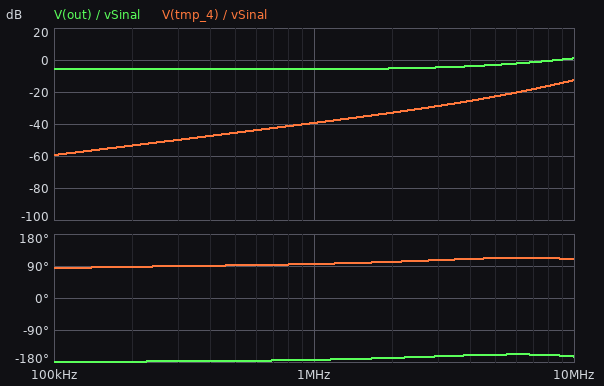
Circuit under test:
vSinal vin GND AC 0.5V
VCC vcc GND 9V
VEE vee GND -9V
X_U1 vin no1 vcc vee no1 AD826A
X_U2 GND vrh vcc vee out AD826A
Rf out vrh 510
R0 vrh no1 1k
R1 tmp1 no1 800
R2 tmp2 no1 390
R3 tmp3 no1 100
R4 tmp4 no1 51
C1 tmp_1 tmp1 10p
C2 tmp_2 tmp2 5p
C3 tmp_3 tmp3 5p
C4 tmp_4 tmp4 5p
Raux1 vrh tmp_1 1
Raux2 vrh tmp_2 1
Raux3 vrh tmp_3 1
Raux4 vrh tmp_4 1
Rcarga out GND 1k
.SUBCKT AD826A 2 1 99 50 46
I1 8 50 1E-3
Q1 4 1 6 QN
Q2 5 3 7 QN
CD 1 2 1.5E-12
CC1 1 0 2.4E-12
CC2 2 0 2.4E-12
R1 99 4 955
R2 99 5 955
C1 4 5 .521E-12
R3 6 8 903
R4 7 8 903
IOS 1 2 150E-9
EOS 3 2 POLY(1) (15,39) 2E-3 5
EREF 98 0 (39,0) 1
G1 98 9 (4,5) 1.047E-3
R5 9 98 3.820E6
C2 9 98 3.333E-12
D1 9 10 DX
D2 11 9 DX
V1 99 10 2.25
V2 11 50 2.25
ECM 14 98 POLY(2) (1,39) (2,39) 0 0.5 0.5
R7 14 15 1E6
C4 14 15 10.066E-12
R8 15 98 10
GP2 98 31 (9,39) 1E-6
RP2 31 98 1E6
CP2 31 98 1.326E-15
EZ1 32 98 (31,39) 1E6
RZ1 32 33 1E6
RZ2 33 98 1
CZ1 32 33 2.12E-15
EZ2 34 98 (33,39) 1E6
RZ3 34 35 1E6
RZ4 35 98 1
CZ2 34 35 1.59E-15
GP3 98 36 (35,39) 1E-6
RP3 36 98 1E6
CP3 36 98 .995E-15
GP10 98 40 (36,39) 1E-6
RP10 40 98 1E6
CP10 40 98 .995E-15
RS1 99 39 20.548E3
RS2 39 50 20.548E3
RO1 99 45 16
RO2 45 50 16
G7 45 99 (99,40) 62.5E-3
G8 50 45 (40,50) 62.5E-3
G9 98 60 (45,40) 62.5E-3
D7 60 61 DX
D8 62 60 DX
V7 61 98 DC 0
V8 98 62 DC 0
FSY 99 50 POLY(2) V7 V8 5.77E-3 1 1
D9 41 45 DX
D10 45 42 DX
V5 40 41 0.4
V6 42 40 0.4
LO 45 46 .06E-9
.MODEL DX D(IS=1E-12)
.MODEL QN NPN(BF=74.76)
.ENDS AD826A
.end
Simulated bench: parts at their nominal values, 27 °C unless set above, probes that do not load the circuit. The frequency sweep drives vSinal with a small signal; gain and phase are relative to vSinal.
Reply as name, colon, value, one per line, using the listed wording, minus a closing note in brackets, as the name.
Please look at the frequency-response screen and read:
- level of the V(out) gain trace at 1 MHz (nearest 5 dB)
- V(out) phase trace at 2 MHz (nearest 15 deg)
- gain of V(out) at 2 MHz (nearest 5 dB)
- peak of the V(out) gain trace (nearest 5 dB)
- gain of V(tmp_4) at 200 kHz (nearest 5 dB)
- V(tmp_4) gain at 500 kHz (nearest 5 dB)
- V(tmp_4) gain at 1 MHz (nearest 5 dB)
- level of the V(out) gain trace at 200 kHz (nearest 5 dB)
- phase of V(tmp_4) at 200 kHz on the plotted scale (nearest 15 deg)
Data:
level of the V(out) gain trace at 1 MHz: -5 dB
V(out) phase trace at 2 MHz: -165 deg
gain of V(out) at 2 MHz: -5 dB
peak of the V(out) gain trace: 0 dB
gain of V(tmp_4) at 200 kHz: -55 dB
V(tmp_4) gain at 500 kHz: -45 dB
V(tmp_4) gain at 1 MHz: -40 dB
level of the V(out) gain trace at 200 kHz: -5 dB
phase of V(tmp_4) at 200 kHz on the plotted scale: 90 deg
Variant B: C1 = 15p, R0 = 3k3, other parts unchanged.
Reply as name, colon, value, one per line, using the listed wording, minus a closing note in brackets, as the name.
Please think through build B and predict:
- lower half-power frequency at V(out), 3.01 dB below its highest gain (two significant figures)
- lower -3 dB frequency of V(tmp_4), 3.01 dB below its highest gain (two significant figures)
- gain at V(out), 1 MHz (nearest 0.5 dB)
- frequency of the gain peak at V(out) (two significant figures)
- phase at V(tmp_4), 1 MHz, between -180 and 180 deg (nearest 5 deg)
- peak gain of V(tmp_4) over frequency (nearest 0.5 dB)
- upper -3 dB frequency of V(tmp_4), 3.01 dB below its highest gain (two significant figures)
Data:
lower half-power frequency at V(out), 3.01 dB below its highest gain: 14 MHz
lower -3 dB frequency of V(tmp_4), 3.01 dB below its highest gain: 19 MHz
gain at V(out), 1 MHz: -14.5 dB
frequency of the gain peak at V(out): 23 MHz
phase at V(tmp_4), 1 MHz, between -180 and 180 deg: 120 deg
peak gain of V(tmp_4) over frequency: 0.5 dB
upper -3 dB frequency of V(tmp_4), 3.01 dB below its highest gain: 71 MHz
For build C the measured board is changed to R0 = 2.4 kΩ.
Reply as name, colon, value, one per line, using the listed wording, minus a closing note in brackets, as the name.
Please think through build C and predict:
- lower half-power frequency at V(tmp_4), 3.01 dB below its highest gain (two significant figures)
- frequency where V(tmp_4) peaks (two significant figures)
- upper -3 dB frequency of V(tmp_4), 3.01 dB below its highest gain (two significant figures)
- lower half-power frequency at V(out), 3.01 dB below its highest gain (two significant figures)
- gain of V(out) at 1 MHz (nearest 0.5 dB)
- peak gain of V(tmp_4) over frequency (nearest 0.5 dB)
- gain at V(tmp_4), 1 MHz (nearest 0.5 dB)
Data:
lower half-power frequency at V(tmp_4), 3.01 dB below its highest gain: 19 MHz
frequency where V(tmp_4) peaks: 28 MHz
upper -3 dB frequency of V(tmp_4), 3.01 dB below its highest gain: 65 MHz
lower half-power frequency at V(out), 3.01 dB below its highest gain: 15 MHz
gain of V(out) at 1 MHz: -13.0 dB
peak gain of V(tmp_4) over frequency: 1.0 dB
gain at V(tmp_4), 1 MHz: -46.5 dB
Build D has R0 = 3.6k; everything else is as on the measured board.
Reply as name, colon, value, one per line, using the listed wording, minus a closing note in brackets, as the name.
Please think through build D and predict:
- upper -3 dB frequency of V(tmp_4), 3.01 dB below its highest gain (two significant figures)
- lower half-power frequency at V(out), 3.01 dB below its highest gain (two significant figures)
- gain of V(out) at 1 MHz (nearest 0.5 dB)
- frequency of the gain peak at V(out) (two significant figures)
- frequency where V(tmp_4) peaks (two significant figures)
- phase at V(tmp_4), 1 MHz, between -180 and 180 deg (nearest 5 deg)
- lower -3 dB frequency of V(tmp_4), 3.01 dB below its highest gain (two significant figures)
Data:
upper -3 dB frequency of V(tmp_4), 3.01 dB below its highest gain: 60 MHz
lower half-power frequency at V(out), 3.01 dB below its highest gain: 15 MHz
gain of V(out) at 1 MHz: -15.5 dB
frequency of the gain peak at V(out): 23 MHz
frequency where V(tmp_4) peaks: 28 MHz
phase at V(tmp_4), 1 MHz, between -180 and 180 deg: 115 deg
lower -3 dB frequency of V(tmp_4), 3.01 dB below its highest gain: 19 MHz
